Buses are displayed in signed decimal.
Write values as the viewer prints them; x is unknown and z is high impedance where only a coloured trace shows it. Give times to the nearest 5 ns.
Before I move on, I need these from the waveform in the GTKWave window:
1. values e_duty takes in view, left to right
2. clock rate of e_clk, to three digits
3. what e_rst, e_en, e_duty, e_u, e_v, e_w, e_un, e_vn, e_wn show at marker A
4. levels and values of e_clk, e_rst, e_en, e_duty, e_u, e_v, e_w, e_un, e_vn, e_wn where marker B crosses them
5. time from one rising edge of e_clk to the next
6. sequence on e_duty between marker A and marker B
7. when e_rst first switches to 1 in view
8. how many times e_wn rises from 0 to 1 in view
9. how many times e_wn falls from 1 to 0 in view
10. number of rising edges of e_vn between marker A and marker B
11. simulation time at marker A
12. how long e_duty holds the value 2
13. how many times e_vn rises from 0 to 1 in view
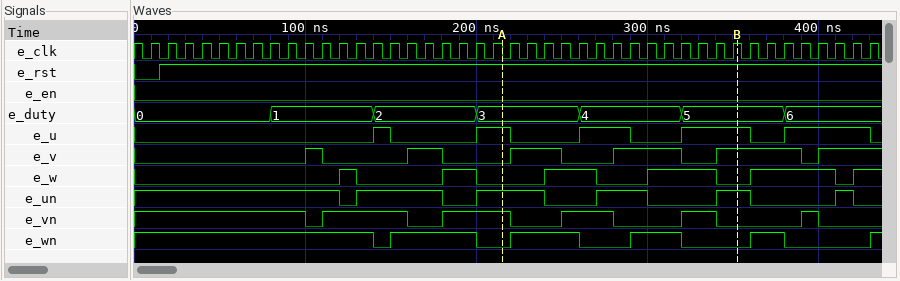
0, 1, 2, 3, 4, 5, 6
100 MHz
e_rst=1, e_en=0, e_duty=3, e_u=1, e_v=0, e_w=0, e_un=1, e_vn=1, e_wn=0
e_clk=1, e_rst=1, e_en=0, e_duty=5, e_u=1, e_v=1, e_w=0, e_un=1, e_vn=0, e_wn=0
10 ns
3, 4, 5
15 ns
5
5
2
215 ns
60 ns
5
